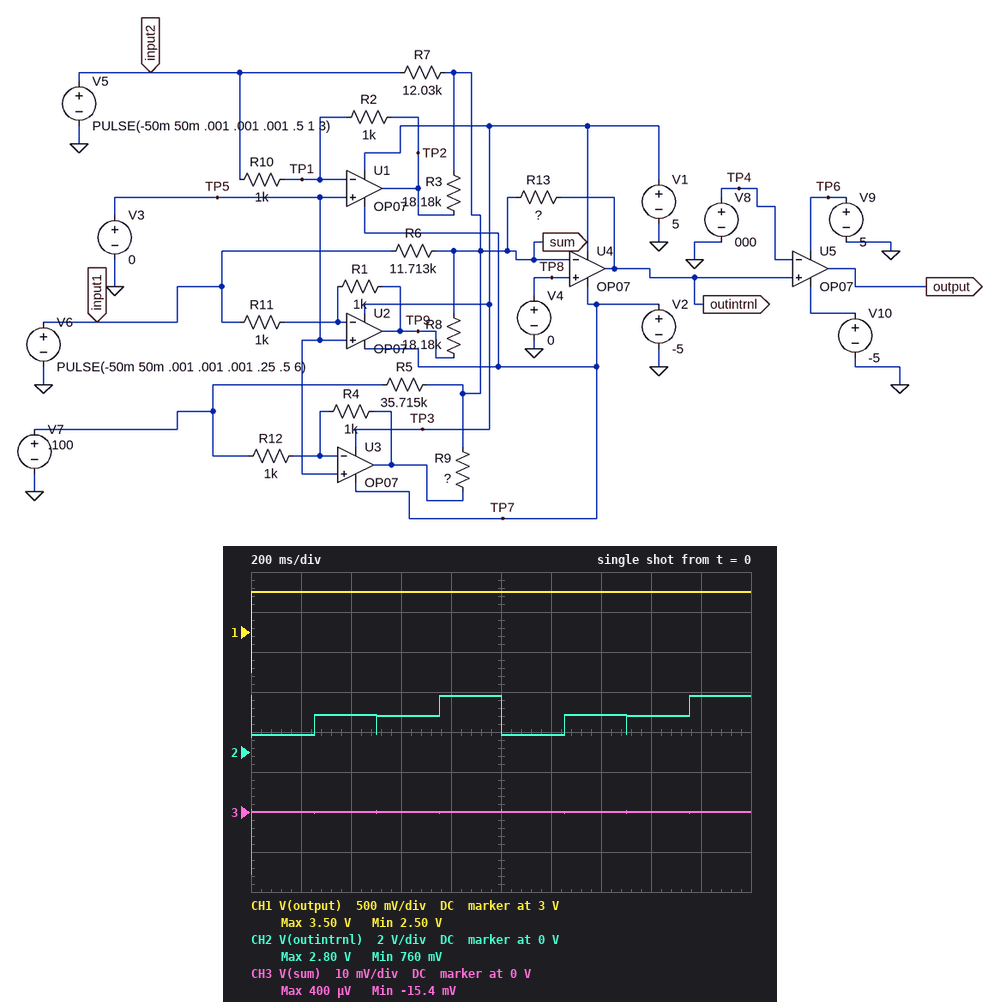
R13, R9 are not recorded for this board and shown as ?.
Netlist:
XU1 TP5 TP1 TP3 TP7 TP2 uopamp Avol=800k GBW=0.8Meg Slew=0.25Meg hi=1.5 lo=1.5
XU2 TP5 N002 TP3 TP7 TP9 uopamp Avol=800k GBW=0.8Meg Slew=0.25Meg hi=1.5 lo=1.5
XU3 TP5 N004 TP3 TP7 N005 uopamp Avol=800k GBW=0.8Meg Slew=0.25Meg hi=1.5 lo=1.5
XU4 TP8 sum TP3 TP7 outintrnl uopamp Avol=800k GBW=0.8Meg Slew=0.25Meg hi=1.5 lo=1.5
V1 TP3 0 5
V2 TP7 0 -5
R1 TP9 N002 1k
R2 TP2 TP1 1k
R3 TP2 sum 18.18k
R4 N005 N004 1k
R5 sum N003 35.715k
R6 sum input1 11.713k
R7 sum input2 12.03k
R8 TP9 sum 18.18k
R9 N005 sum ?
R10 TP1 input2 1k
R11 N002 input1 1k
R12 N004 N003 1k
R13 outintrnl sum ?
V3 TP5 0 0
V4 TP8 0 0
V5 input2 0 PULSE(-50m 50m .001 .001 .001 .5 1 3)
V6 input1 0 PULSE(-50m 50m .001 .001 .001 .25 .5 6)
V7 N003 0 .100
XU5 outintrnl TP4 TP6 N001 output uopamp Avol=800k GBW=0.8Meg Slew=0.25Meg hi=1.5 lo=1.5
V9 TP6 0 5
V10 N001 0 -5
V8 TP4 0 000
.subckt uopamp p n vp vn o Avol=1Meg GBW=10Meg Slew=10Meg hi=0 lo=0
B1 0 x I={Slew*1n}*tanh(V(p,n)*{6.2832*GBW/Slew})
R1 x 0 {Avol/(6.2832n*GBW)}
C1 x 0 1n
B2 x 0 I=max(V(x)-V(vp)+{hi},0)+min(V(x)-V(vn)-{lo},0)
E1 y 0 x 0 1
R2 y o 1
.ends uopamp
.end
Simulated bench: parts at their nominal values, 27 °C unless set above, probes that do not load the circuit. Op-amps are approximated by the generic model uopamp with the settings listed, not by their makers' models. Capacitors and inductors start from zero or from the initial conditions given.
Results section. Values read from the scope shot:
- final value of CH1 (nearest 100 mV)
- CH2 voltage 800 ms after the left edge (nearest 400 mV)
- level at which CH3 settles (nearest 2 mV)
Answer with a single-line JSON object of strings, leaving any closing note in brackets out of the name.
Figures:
{"final value of CH1": "3.5 V", "CH2 voltage 800 ms after the left edge": "2.8 V", "level at which CH3 settles": "0 V"}
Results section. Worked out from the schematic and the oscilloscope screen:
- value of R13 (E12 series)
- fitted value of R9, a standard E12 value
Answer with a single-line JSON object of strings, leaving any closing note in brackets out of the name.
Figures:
{"value of R13": "330 kΩ", "fitted value of R9, a standard E12 value": "12 kΩ"}
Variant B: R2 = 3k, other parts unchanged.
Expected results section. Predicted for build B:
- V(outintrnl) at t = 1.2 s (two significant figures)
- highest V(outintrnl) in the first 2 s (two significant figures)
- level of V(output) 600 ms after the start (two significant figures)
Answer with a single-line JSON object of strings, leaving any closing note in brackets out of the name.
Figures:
{"V(outintrnl) at t = 1.2 s": "2.7 V", "highest V(outintrnl) in the first 2 s": "3.5 V", "level of V(output) 600 ms after the start": "-3.5 V"}
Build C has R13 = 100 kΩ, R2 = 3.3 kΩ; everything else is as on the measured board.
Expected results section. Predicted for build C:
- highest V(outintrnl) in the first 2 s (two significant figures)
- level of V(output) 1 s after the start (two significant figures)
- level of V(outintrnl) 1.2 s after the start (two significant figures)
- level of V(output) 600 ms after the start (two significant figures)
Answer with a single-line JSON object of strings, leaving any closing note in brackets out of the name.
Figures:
{"highest V(outintrnl) in the first 2 s": "1.2 V", "level of V(output) 1 s after the start": "3.5 V", "level of V(outintrnl) 1.2 s after the start": "890 mV", "level of V(output) 600 ms after the start": "-3.5 V"}
